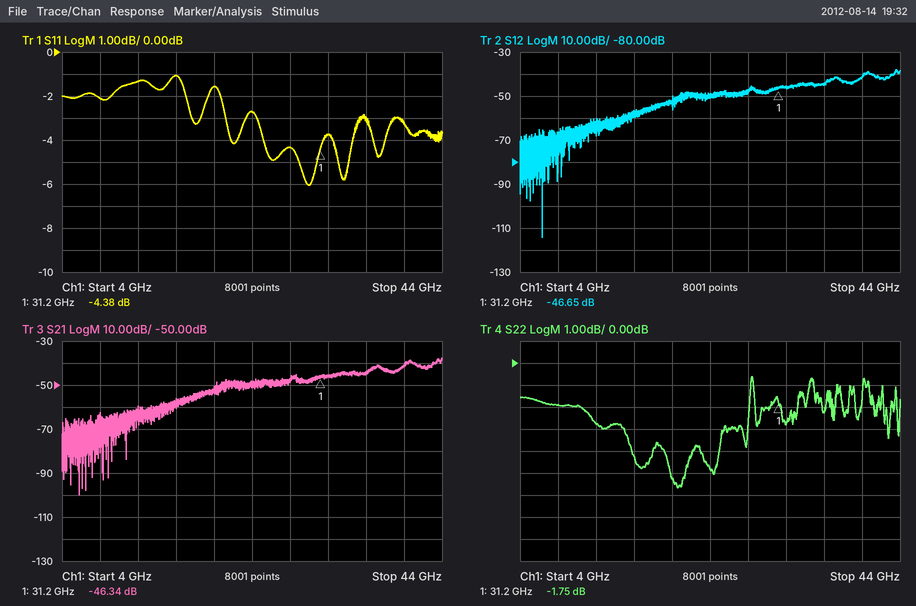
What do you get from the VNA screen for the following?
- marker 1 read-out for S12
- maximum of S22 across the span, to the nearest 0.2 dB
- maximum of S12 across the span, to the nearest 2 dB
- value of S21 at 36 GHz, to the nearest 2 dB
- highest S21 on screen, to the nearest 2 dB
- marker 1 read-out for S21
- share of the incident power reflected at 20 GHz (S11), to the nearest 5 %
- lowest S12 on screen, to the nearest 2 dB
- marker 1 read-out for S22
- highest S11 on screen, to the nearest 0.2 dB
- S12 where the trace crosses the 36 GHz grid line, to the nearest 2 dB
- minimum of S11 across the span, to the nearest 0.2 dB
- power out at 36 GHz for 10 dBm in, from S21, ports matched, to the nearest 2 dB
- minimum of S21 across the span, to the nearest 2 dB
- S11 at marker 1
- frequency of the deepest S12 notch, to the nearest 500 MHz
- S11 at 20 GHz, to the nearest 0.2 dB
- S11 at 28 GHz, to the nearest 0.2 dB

-46.65 dB
-0.6 dB
-38 dB
-44 dB
-38 dB
-46.34 dB
70 %
-114 dB
-1.75 dB
-1.0 dB
-44 dB
-6.0 dB
-34 dBm
-100 dB
-4.38 dB
6.5 GHz
-1.6 dB
-4.4 dB
